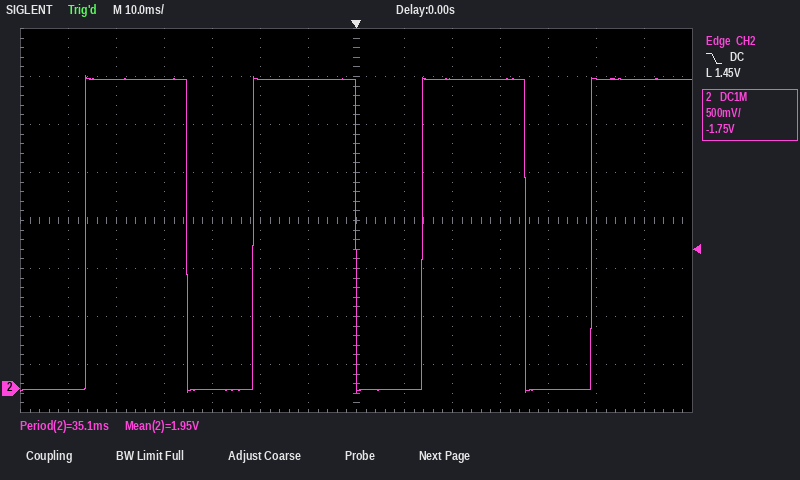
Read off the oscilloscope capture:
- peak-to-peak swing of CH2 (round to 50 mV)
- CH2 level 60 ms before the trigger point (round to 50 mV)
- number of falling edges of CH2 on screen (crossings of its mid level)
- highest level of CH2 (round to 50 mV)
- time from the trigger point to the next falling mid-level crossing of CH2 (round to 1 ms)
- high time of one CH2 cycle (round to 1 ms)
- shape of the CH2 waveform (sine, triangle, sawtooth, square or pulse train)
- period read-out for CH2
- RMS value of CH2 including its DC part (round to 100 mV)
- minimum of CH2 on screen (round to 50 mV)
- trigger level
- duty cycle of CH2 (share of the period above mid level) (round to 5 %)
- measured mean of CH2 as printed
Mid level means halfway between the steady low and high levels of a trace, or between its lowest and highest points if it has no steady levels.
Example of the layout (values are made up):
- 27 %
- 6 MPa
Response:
- 3.30 V
- 0 mV
- 3
- 3.25 V
- 35 ms
- 21 ms
- pulse train
- 35.1 ms
- 2.5 V
- -50 mV
- 1.45 V
- 60 %
- 1.95 V
